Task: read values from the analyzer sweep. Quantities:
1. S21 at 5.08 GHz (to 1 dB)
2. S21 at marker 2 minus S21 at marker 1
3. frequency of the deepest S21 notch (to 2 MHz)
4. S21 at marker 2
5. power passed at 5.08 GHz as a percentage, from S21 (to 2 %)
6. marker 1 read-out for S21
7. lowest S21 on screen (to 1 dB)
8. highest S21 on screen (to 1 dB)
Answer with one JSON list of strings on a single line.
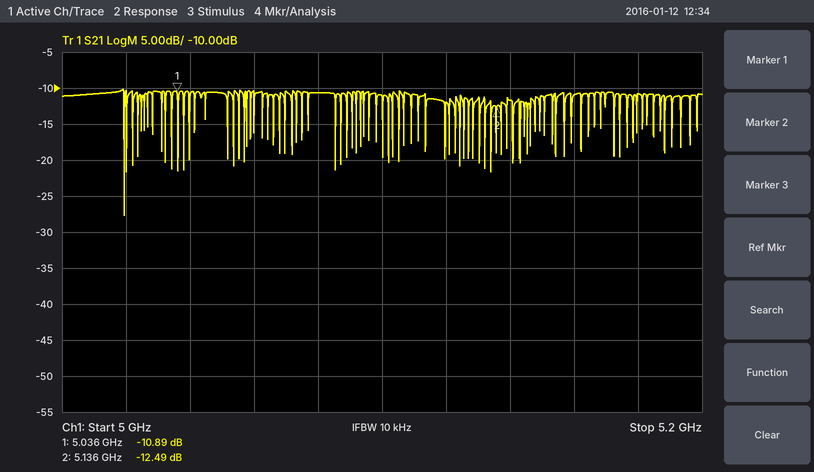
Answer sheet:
["-11 dB", "-1.60 dB", "5.020 GHz", "-12.49 dB", "8 %", "-10.89 dB", "-28 dB", "-10 dB"]
